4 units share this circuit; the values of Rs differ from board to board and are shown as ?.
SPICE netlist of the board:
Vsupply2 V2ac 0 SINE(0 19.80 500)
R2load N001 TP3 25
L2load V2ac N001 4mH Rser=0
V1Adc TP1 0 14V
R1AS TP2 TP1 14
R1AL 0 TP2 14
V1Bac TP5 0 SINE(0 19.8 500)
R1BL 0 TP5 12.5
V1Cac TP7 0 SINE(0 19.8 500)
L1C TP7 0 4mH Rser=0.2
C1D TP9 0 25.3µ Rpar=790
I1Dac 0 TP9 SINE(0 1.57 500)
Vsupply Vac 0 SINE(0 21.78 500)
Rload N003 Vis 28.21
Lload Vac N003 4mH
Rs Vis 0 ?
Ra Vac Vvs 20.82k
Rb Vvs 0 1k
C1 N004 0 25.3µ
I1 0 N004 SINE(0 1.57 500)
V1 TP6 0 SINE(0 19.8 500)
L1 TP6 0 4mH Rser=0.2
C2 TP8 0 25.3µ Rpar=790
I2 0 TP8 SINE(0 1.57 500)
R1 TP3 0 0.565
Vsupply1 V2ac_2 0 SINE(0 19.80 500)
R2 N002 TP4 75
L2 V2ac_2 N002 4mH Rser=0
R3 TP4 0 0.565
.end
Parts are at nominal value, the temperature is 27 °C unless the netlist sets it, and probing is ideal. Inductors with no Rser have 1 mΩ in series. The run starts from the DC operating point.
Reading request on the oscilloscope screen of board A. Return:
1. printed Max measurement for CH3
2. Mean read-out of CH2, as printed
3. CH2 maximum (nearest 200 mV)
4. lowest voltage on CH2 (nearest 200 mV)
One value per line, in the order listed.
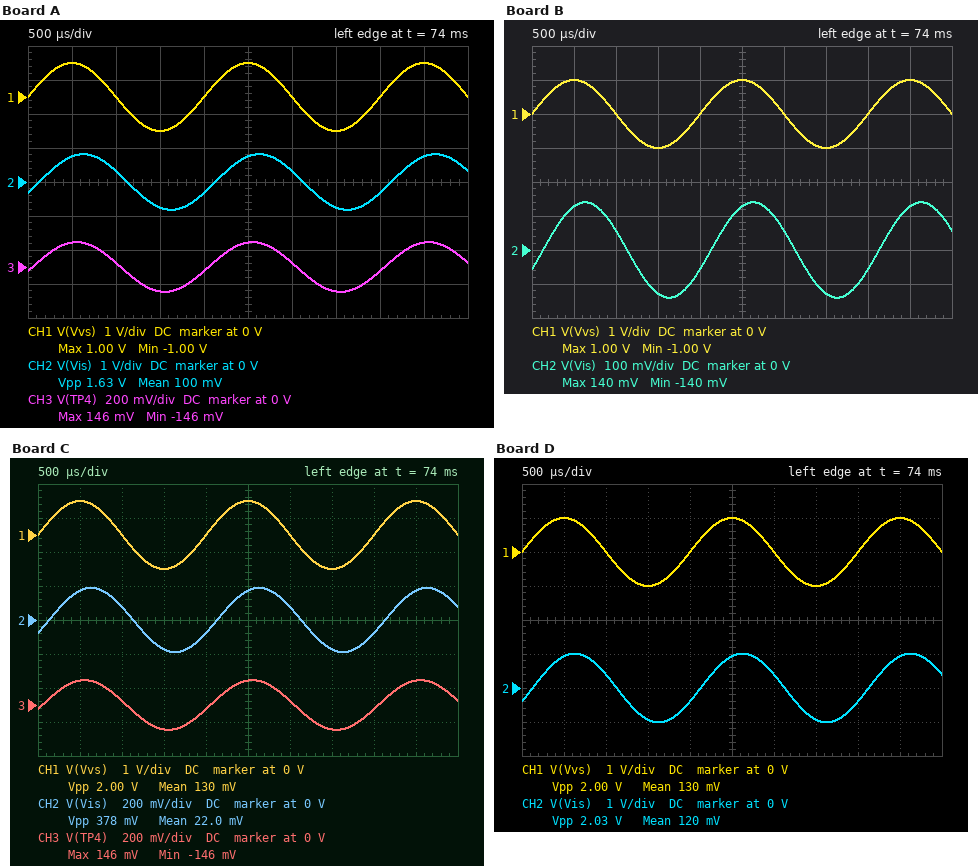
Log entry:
146 mV
100 mV
800 mV
-800 mV
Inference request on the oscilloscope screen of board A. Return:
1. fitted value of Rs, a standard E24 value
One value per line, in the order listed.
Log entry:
1.2 Ω
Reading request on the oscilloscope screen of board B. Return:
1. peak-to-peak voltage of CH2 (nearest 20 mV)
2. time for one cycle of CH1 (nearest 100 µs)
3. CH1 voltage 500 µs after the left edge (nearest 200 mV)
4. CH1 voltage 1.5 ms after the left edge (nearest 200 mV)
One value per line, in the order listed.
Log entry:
280 mV
2.0 ms
1.0 V
-1.0 V
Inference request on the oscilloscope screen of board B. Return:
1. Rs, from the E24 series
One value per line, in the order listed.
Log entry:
0.2 Ω
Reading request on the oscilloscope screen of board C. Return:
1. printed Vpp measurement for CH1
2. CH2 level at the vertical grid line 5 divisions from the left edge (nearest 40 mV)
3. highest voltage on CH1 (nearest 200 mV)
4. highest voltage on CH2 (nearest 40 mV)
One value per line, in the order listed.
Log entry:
2.00 V
160 mV
1.0 V
200 mV
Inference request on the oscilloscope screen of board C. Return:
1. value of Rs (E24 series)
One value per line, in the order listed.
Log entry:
0.27 Ω
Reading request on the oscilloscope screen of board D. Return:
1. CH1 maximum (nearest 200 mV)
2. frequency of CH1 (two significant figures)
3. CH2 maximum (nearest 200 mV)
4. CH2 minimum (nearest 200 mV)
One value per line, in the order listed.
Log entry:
1.0 V
500 Hz
1.0 V
-1.0 V
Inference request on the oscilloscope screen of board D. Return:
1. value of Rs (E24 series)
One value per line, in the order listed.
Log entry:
1.5 Ω
